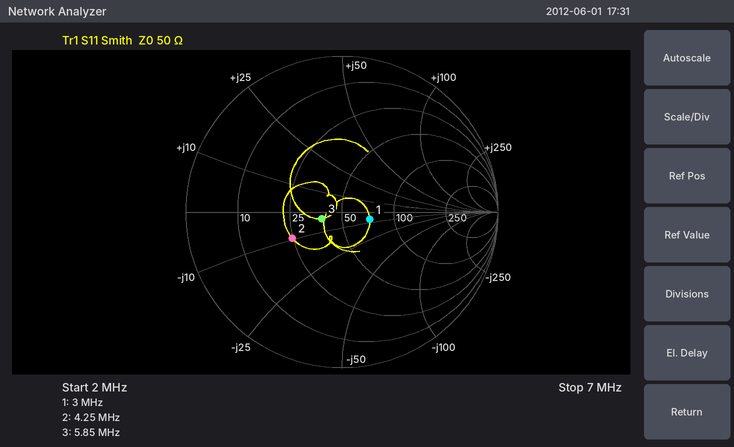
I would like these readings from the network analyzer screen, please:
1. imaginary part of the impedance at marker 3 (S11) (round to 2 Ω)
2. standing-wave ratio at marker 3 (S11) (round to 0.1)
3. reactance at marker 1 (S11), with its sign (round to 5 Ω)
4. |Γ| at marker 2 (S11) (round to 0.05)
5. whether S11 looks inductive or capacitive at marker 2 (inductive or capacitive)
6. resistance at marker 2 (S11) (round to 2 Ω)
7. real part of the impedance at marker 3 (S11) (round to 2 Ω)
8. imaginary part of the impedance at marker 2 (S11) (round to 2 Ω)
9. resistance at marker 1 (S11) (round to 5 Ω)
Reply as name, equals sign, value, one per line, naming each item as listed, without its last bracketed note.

imaginary part of the impedance at marker 3 (S11) = -4 Ω
standing-wave ratio at marker 3 (S11) = 1.3
reactance at marker 1 (S11), with its sign = -5 Ω
|Γ| at marker 2 (S11) = 0.35
whether S11 looks inductive or capacitive at marker 2 = capacitive
resistance at marker 2 (S11) = 24 Ω
real part of the impedance at marker 3 (S11) = 38 Ω
imaginary part of the impedance at marker 2 (S11) = -10 Ω
resistance at marker 1 (S11) = 70 Ω
